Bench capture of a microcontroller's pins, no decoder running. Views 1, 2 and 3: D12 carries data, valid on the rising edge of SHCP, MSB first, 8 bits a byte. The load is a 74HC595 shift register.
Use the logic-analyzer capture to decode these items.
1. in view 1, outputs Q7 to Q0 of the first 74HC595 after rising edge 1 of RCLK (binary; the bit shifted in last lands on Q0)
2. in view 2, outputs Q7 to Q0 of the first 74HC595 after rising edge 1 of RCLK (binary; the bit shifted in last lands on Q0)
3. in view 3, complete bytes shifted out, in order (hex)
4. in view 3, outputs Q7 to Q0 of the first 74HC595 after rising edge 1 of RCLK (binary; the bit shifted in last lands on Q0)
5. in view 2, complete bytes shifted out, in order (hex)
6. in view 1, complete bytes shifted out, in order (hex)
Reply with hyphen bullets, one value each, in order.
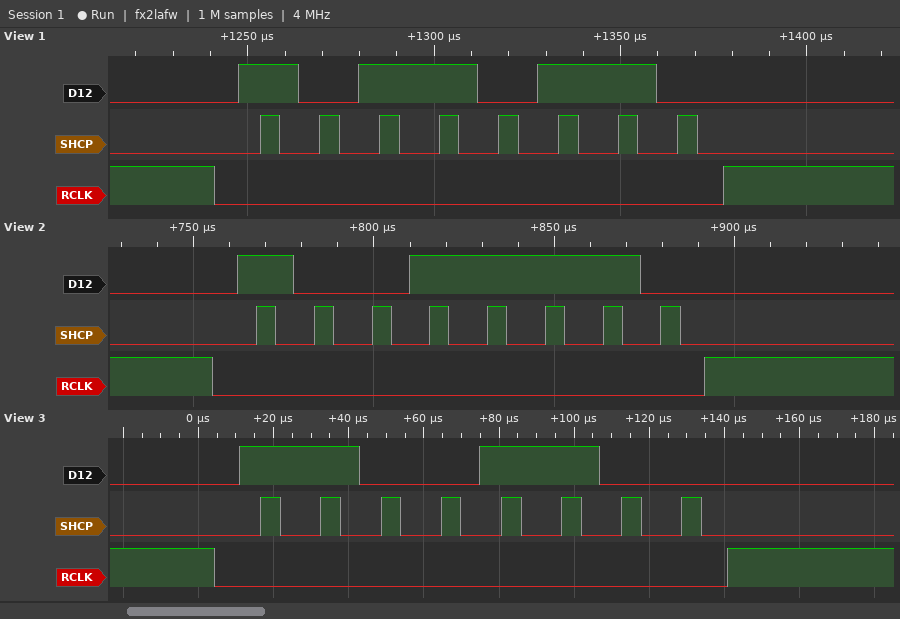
- 10110110
- 10011110
- CC
- 11001100
- 9E
- B6
